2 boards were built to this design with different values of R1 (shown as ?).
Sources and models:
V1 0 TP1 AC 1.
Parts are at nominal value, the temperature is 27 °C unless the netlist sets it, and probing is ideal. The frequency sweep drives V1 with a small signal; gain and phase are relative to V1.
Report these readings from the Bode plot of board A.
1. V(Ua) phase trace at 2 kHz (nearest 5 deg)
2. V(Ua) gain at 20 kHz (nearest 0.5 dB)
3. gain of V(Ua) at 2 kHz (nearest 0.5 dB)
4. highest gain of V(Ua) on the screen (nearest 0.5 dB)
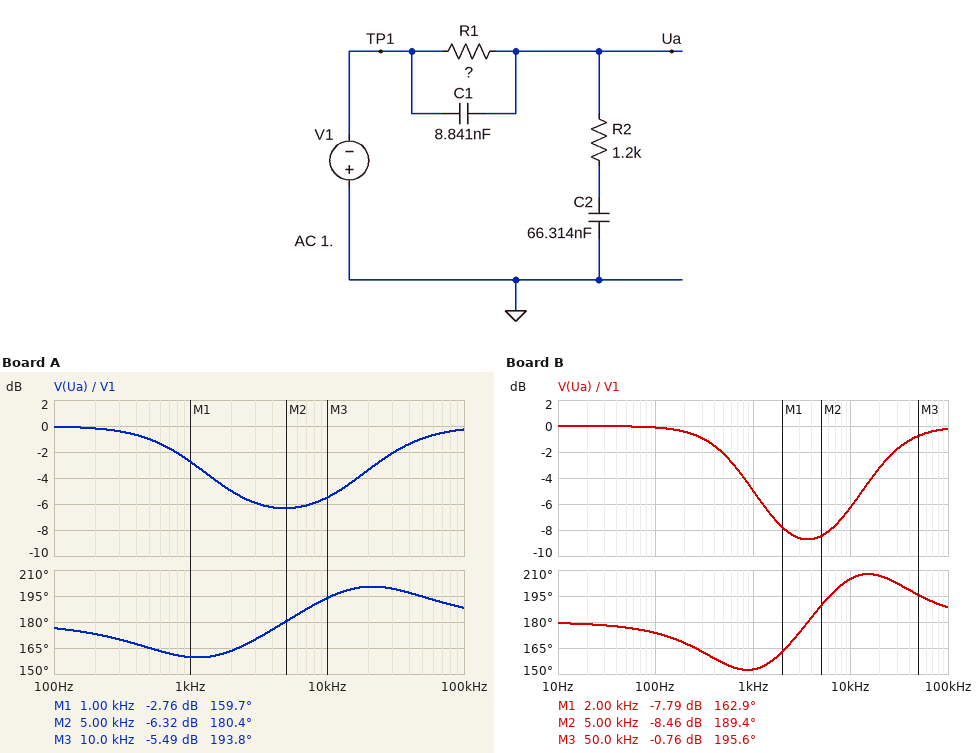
165 deg
-3.5 dB
-5.0 dB
0 dB
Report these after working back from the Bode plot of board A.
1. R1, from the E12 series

1.5 kΩ
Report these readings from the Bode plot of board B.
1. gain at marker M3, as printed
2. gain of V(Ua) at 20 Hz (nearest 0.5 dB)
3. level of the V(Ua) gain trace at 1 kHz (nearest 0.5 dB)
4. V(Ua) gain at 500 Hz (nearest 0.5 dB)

-0.76 dB
0 dB
-5.0 dB
-2.0 dB
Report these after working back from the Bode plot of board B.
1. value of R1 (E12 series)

2.7 kΩ
